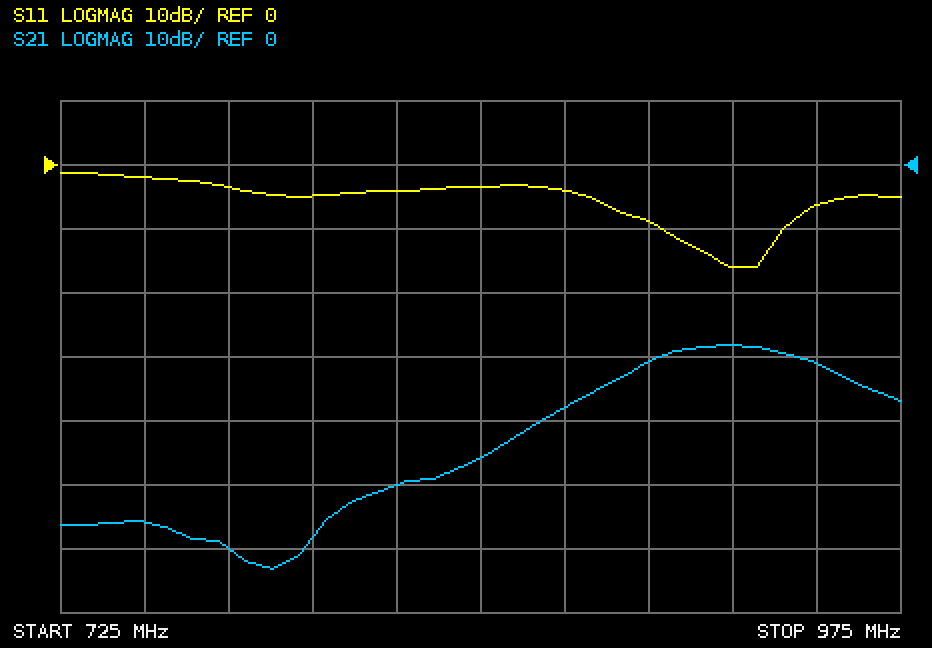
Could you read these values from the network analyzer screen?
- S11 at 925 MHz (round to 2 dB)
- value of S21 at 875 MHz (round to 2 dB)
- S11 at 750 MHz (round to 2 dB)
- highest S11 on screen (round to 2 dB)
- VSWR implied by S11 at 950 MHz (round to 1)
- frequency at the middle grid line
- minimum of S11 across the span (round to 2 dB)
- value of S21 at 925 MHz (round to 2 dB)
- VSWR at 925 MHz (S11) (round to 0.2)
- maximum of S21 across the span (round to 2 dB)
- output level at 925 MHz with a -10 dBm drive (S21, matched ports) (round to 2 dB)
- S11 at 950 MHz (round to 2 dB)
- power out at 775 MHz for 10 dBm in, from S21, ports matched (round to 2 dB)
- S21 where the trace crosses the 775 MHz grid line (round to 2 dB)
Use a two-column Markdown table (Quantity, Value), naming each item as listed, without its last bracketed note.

| Quantity | Value |
|---|---|
| S11 at 925 MHz | -16 dB |
| value of S21 at 875 MHz | -38 dB |
| S11 at 750 MHz | -2 dB |
| highest S11 on screen | -2 dB |
| VSWR implied by S11 at 950 MHz | 3 |
| frequency at the middle grid line | 850 MHz |
| minimum of S11 across the span | -16 dB |
| value of S21 at 925 MHz | -28 dB |
| VSWR at 925 MHz (S11) | 1.4 |
| maximum of S21 across the span | -28 dB |
| output level at 925 MHz with a -10 dBm drive (S21, matched ports) | -38 dBm |
| S11 at 950 MHz | -6 dB |
| power out at 775 MHz for 10 dBm in, from S21, ports matched | -50 dBm |
| S21 where the trace crosses the 775 MHz grid line | -60 dB |
